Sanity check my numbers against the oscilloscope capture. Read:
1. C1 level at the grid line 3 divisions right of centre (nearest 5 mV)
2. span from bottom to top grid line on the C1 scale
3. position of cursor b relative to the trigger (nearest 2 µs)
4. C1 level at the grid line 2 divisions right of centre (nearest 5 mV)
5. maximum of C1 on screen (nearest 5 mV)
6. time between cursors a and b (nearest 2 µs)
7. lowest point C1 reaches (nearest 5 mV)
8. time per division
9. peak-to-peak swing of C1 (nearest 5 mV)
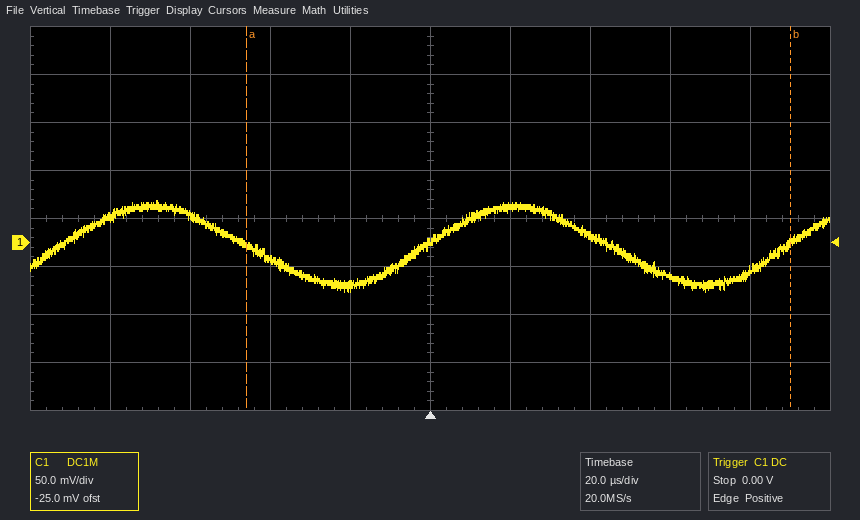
-35 mV
400 mV
+90 µs
5 mV
45 mV
136 µs
-50 mV
20 µs
95 mV
